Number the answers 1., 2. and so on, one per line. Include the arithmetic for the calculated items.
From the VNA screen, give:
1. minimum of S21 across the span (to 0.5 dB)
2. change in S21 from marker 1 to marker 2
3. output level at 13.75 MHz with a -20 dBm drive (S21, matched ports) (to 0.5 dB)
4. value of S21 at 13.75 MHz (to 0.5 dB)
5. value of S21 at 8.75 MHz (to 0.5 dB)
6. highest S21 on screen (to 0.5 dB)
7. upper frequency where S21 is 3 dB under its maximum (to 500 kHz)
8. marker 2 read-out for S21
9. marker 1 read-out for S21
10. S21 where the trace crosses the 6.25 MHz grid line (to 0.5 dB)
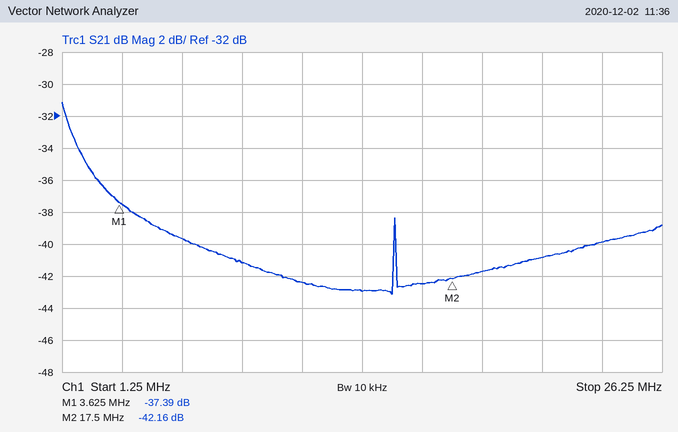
1. -43.0 dB
2. -42.16 − (-37.39) = -4.77 dB
3. -20 dBm + (-43.0 dB) = -63.0 dBm
4. -43.0 dB
5. -41.0 dB
6. -31.0 dB
7. 2.0 MHz
8. -42.16 dB
9. -37.39 dB
10. -39.5 dB
